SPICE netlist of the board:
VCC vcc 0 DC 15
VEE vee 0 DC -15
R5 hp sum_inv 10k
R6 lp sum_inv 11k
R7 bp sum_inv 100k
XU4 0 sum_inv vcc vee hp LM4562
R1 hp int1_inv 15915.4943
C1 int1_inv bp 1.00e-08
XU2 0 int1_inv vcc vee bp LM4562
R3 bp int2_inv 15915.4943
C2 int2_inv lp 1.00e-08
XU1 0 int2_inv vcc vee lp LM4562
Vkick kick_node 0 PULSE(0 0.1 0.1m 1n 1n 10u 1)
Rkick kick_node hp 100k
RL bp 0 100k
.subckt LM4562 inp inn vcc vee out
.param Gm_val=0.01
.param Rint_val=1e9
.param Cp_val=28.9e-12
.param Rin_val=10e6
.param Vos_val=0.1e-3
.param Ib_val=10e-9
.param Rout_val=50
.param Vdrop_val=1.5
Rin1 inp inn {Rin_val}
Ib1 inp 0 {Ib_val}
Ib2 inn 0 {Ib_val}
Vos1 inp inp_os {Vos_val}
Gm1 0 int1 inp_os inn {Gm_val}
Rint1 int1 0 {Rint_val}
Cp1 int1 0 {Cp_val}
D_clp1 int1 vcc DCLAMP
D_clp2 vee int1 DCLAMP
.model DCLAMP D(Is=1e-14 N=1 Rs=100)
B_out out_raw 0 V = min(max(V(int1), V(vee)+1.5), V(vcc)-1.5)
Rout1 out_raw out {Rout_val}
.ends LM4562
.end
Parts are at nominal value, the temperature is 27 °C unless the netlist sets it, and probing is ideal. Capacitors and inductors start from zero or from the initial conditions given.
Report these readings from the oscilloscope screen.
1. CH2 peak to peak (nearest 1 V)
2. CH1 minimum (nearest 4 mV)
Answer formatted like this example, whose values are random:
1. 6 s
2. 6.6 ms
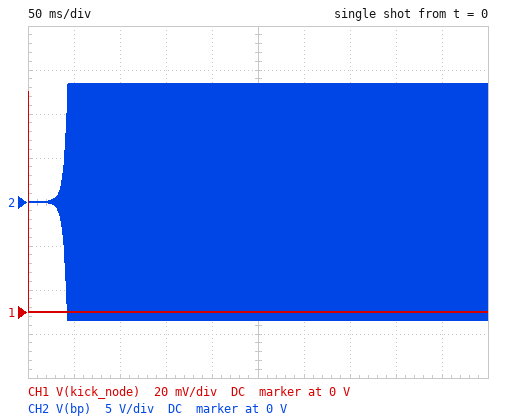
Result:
1. 27 V
2. 0 V
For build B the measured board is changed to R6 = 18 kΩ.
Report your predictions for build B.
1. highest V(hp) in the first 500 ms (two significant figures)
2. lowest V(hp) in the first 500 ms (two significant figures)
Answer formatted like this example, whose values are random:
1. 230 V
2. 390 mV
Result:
1. 8.0 V
2. -8.0 V
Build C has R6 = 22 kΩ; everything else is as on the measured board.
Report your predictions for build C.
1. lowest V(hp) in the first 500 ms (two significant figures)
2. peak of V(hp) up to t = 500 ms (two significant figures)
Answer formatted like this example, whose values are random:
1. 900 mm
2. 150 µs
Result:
1. -6.6 V
2. 6.6 V
